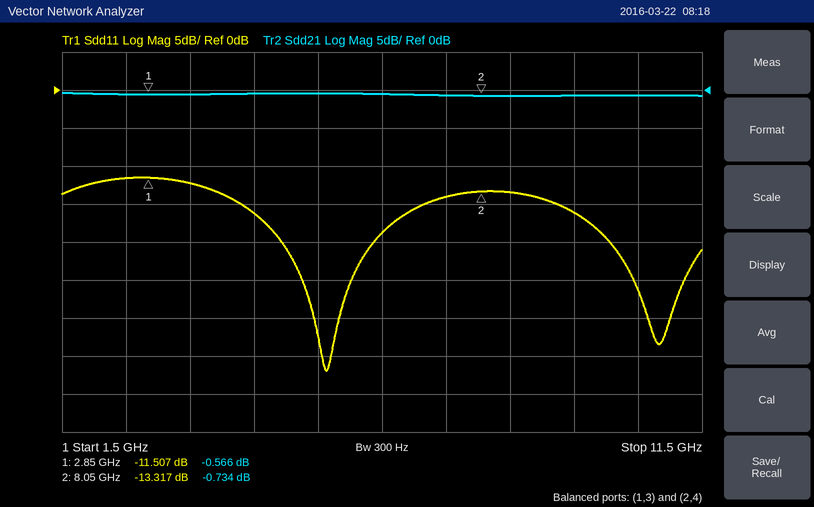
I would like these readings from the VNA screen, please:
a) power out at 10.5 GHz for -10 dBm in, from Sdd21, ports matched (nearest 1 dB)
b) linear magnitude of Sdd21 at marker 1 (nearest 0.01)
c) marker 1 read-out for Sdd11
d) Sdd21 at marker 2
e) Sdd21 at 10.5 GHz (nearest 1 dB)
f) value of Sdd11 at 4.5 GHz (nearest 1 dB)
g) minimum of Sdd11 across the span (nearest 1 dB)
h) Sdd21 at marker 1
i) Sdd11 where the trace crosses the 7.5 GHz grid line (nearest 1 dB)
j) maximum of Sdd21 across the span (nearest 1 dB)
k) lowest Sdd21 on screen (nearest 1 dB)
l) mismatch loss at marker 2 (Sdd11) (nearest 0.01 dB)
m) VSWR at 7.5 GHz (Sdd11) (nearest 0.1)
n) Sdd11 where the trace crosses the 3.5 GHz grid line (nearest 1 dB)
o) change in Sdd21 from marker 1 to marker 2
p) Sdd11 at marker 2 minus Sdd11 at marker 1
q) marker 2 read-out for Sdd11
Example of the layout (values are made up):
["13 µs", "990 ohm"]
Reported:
["-11 dBm", "0.94", "-11.507 dB", "-0.734 dB", "-1 dB", "-16 dB", "-37 dB", "-0.566 dB", "-14 dB", "0 dB", "-1 dB", "0.21 dB", "1.5", "-12 dB", "-0.168 dB", "-1.810 dB", "-13.317 dB"]
